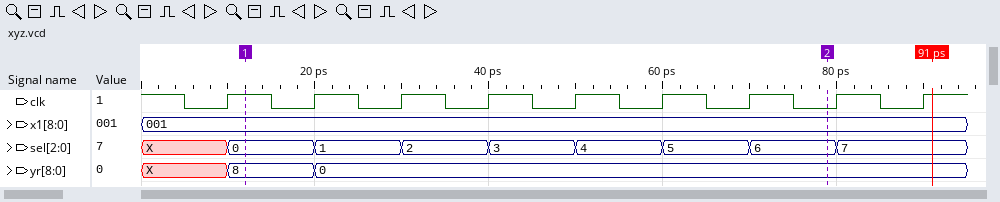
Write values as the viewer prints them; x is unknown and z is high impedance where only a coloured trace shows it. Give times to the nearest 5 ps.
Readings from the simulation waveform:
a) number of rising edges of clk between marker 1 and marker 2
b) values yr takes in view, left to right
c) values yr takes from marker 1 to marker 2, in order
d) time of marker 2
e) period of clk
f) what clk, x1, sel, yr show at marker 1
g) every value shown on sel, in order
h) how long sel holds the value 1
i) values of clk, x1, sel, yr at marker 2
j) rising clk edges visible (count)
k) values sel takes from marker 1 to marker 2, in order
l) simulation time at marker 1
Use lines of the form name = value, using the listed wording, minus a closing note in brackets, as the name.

number of rising edges of clk between marker 1 and marker 2 = 6
values yr takes in view, left to right = X, 8, 0
values yr takes from marker 1 to marker 2, in order = 8, 0
time of marker 2 = 80 ps
period of clk = 10 ps
what clk, x1, sel, yr show at marker 1 = clk=1, x1=001, sel=0, yr=8
every value shown on sel, in order = X, 0, 1, 2, 3, 4, 5, 6, 7
how long sel holds the value 1 = 10 ps
values of clk, x1, sel, yr at marker 2 = clk=0, x1=001, sel=6, yr=0
rising clk edges visible = 9
values sel takes from marker 1 to marker 2, in order = 0, 1, 2, 3, 4, 5, 6
simulation time at marker 1 = 10 ps
